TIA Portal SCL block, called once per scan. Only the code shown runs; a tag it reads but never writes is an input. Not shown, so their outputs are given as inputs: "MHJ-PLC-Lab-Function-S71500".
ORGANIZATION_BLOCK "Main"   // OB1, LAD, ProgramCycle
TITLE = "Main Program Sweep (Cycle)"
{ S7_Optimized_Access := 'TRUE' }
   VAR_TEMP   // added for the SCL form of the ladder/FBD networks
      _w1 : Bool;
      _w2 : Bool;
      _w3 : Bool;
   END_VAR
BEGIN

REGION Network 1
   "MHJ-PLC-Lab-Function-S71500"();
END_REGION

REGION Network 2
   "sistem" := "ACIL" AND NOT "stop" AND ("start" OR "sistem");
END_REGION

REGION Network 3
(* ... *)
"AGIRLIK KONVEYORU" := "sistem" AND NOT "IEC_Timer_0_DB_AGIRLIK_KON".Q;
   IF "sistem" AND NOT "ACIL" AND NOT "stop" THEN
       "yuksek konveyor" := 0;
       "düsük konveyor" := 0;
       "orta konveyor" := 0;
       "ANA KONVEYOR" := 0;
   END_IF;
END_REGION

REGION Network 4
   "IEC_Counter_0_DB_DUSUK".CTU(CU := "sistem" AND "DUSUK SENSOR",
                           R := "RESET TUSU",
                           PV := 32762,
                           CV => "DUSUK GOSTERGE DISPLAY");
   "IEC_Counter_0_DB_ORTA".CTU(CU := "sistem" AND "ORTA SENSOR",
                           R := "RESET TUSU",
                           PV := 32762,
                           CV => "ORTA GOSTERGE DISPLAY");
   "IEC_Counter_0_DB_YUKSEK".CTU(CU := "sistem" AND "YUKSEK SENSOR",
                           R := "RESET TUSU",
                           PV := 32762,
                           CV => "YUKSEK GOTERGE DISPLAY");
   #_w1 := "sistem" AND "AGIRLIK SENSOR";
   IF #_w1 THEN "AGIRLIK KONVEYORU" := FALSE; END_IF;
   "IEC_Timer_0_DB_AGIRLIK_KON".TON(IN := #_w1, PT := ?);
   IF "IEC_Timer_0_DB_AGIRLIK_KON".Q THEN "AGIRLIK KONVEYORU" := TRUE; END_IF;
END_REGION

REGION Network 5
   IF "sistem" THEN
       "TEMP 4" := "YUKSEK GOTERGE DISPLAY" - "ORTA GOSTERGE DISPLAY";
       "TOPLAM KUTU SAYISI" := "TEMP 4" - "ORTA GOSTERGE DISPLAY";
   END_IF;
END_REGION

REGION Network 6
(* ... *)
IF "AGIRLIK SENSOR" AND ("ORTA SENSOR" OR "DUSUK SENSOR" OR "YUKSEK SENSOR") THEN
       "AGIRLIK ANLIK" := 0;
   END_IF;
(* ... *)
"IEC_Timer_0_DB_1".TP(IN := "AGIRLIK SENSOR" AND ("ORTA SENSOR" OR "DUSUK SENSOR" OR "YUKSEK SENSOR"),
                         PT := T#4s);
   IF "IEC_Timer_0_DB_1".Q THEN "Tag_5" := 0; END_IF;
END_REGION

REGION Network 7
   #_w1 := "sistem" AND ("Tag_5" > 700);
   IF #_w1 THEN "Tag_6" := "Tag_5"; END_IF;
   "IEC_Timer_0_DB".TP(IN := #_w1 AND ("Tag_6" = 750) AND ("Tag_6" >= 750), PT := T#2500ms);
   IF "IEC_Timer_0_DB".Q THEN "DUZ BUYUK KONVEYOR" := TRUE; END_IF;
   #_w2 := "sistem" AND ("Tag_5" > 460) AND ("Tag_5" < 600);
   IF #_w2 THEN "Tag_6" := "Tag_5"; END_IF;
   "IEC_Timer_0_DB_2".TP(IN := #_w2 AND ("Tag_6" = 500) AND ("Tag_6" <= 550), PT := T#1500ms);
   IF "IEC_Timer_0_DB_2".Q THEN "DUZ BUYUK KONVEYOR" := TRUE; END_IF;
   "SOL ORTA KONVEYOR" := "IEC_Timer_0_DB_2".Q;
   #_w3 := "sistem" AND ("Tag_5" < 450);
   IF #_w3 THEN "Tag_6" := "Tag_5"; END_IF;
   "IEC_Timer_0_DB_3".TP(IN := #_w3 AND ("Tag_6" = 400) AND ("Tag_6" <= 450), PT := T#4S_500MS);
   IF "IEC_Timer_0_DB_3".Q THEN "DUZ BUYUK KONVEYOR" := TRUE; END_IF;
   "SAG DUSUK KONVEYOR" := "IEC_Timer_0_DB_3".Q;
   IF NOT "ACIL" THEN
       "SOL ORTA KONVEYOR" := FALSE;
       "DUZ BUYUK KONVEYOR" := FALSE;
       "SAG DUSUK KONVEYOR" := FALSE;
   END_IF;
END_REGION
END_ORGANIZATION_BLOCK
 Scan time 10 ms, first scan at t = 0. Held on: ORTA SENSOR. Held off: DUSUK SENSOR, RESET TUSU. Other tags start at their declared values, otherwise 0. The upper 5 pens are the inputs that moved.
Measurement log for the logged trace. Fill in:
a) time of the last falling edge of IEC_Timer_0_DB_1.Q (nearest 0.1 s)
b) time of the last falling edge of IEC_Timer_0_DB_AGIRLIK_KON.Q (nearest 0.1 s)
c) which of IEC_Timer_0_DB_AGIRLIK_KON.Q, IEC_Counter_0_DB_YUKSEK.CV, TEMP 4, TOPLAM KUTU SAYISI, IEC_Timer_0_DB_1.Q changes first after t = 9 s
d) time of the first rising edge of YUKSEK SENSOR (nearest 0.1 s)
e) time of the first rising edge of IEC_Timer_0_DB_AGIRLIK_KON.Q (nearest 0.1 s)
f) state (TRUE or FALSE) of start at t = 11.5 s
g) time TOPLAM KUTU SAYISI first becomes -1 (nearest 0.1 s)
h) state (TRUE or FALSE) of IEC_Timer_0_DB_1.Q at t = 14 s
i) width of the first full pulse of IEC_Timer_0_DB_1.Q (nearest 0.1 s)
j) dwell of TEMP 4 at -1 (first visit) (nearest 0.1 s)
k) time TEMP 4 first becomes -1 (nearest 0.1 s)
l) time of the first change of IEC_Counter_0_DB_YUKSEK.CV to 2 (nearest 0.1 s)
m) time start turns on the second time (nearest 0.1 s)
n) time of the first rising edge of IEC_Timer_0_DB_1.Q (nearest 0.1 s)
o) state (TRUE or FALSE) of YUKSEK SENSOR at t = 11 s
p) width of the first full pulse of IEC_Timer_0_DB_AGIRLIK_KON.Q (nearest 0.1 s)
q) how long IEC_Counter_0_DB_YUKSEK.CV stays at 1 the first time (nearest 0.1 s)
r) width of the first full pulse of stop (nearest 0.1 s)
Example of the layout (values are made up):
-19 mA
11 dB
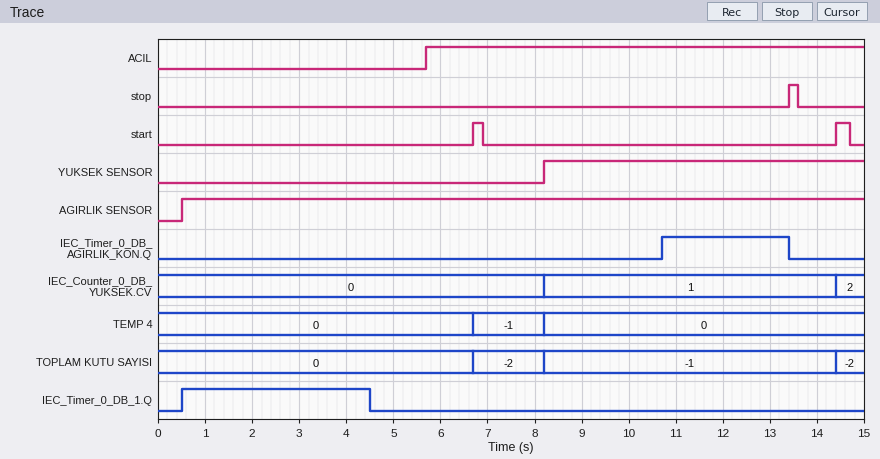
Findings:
4.5 s
13.4 s
IEC_Timer_0_DB_AGIRLIK_KON.Q
8.2 s
10.7 s
FALSE
8.2 s
FALSE
4.0 s
1.5 s
6.7 s
14.4 s
14.4 s
0.5 s
TRUE
2.7 s
6.2 s
0.2 s
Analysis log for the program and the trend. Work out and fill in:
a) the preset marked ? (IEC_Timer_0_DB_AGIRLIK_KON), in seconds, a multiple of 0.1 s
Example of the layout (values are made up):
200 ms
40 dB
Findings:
4.0 s
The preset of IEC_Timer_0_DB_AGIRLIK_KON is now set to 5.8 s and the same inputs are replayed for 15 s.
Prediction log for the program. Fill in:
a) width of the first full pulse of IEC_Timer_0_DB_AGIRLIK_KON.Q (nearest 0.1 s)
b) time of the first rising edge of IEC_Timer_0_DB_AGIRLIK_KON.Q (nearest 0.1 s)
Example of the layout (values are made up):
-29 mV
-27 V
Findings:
0.9 s
12.5 s
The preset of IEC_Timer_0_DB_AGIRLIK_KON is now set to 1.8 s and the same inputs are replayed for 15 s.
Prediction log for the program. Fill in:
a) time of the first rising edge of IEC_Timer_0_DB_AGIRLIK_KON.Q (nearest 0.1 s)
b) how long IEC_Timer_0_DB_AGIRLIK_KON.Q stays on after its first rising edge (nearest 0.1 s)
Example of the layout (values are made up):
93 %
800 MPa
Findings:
8.5 s
4.9 s
